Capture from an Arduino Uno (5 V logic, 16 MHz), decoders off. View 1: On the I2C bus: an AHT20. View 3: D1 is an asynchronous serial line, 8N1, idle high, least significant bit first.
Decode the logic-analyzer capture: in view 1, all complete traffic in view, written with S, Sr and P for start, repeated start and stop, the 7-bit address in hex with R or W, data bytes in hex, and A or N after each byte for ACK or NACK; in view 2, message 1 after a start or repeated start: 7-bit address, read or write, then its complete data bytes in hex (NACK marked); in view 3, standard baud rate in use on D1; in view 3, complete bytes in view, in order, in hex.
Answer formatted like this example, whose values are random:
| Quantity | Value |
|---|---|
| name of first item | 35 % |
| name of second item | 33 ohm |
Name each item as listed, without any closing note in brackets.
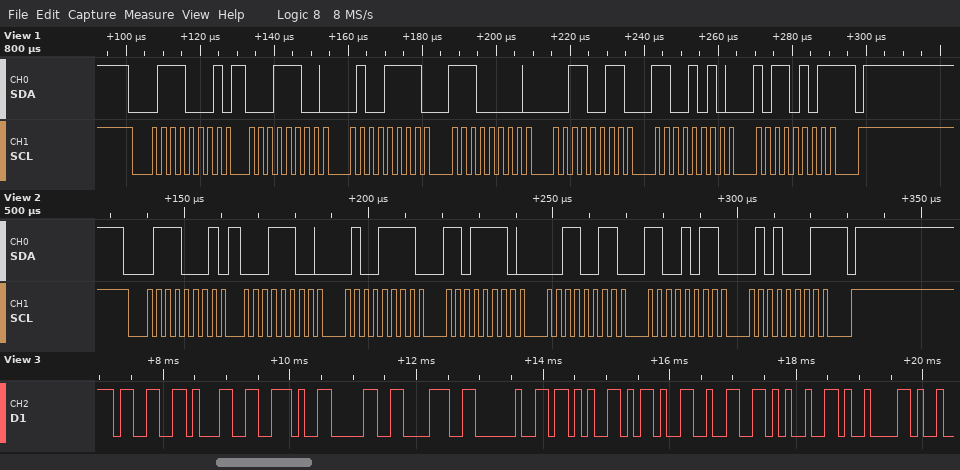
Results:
| Quantity | Value |
|---|---|
| in view 1, all complete traffic in view, written with S, Sr and P for start, repeated start and stop, the 7-bit address in hex with R or W, data bytes in hex, and A or N after each byte for ACK or NACK | S 38R A 1C A 4F A E0 A 33 A CA A B5 N P |
| in view 2, message 1 after a start or repeated start: 7-bit address, read or write, then its complete data bytes in hex | 0x38 read: 1C 4F DE 33 CB 51 NACK |
| in view 3, standard baud rate in use on D1 | 9600 baud |
| in view 3, complete bytes in view, in order, in hex | 33 31 2E 30 38 20 2B 2D 32 25 09 |
